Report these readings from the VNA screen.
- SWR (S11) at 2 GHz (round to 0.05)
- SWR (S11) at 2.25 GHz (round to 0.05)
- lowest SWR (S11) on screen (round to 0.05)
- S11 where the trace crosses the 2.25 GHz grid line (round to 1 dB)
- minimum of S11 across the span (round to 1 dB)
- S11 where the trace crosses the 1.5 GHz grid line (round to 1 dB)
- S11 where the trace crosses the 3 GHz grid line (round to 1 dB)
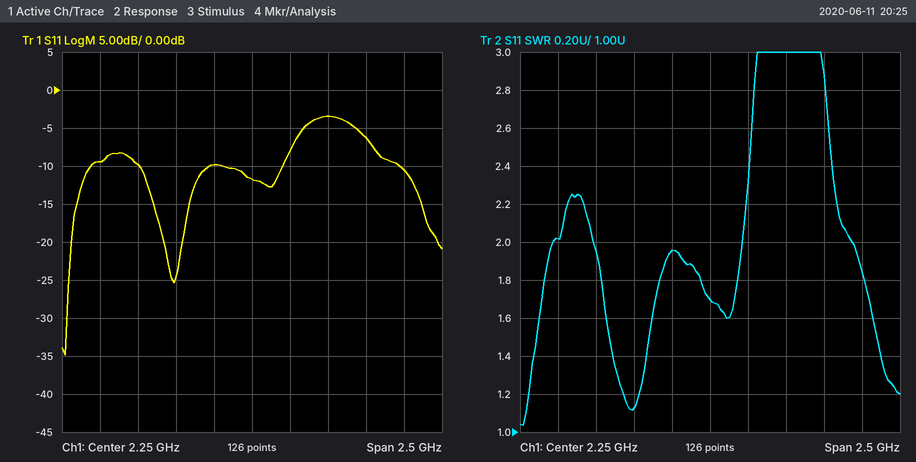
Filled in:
1.95
1.70
1.05
-12 dB
-35 dB
-10 dB
-6 dB
